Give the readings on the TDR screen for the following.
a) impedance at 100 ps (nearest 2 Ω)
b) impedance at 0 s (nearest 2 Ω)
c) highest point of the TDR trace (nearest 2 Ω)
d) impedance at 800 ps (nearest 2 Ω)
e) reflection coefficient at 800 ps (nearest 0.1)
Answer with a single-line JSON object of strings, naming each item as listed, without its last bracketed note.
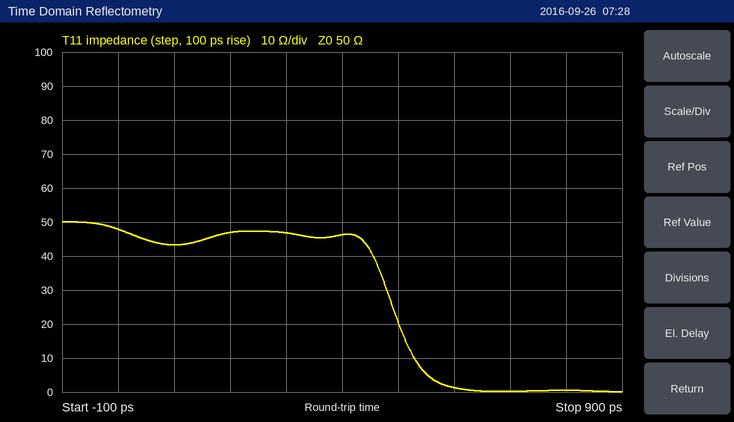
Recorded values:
{"impedance at 100 ps": "44 Ω", "impedance at 0 s": "48 Ω", "highest point of the TDR trace": "50 Ω", "impedance at 800 ps": "0 Ω", "reflection coefficient at 800 ps": "-1.0"}
